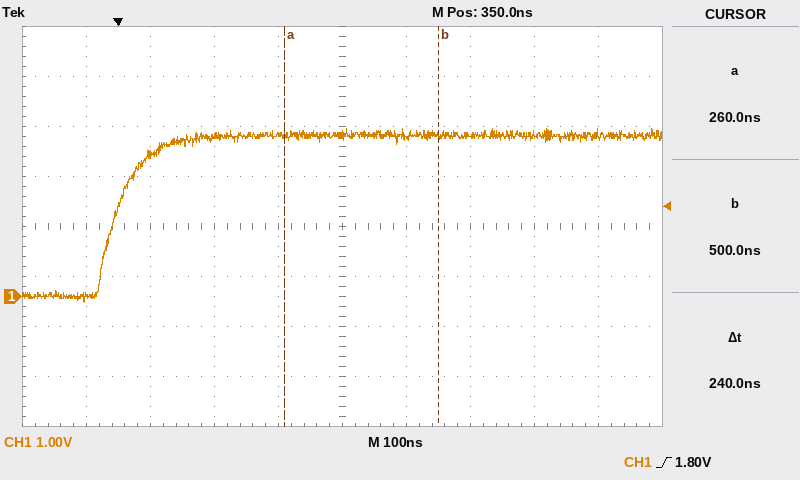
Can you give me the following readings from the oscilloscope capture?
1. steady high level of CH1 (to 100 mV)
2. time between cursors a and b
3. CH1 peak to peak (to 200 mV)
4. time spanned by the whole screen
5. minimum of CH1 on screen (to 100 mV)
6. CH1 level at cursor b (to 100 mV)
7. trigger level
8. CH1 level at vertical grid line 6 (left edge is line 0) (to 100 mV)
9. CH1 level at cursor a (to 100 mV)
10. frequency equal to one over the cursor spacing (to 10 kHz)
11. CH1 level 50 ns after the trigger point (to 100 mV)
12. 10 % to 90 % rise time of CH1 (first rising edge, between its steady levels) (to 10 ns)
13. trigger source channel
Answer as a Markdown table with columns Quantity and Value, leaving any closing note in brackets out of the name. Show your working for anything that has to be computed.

| Quantity | Value |
|---|---|
| steady high level of CH1 | 3.2 V |
| time between cursors a and b | 240 ns |
| CH1 peak to peak | 3.4 V |
| time spanned by the whole screen | 1 µs |
| minimum of CH1 on screen | -100 mV |
| CH1 level at cursor b | 3.2 V |
| trigger level | 1.80 V |
| CH1 level at vertical grid line 6 (left edge is line 0) | 3.2 V |
| CH1 level at cursor a | 3.2 V |
| frequency equal to one over the cursor spacing | 1 / 240 ns ≈ 4.17 MHz |
| CH1 level 50 ns after the trigger point | 2.8 V |
| 10 % to 90 % rise time of CH1 (first rising edge, between its steady levels) | 90 ns |
| trigger source channel | CH1 |
